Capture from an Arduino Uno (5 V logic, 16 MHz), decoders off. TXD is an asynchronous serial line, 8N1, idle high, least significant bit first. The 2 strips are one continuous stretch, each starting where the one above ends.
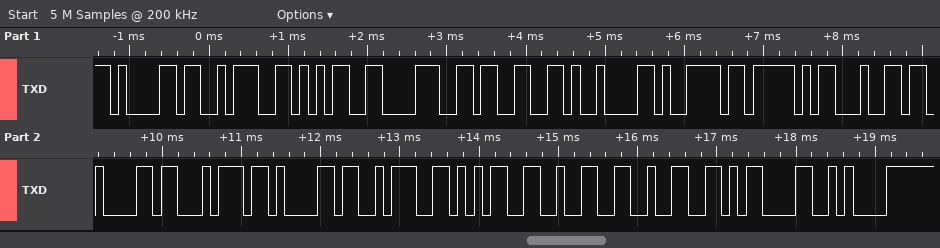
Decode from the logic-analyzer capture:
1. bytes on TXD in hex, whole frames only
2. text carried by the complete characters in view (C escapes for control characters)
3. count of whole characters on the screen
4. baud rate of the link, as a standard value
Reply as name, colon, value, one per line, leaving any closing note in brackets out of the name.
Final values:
bytes on TXD in hex, whole frames only: 61 3A 35 38 33 09 79 5F 64 61 74 61 3A 35 32 32 0D 0A
text carried by the complete characters in view: "a:583\ty_data:522\r\n"
count of whole characters on the screen: 18
baud rate of the link, as a standard value: 9600 baud
